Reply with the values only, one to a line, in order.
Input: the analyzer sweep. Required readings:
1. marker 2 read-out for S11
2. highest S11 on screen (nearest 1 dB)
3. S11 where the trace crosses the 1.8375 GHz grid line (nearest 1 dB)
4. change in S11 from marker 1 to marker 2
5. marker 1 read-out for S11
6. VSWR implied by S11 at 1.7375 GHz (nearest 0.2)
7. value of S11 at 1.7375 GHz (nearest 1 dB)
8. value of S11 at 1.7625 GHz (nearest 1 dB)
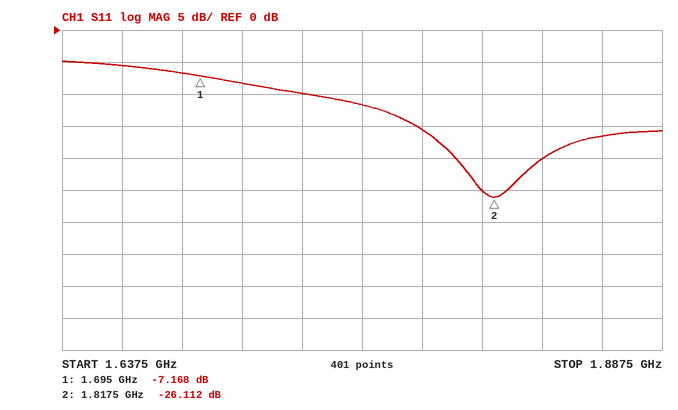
-26.112 dB
-5 dB
-20 dB
-18.944 dB
-7.168 dB
2.0
-10 dB
-12 dB
